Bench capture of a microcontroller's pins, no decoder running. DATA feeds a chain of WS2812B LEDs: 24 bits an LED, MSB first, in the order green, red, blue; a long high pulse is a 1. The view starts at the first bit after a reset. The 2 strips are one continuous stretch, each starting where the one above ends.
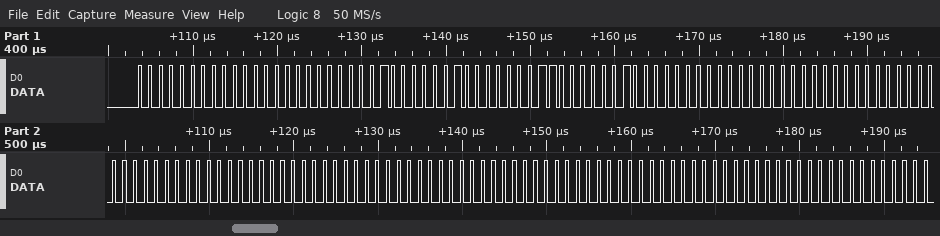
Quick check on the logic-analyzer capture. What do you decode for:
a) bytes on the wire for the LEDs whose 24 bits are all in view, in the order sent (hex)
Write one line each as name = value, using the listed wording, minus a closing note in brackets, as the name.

bytes on the wire for the LEDs whose 24 bits are all in view, in the order sent = 00 00 01 02 03 02 00 00 00 00 00 00 00 00 00 00 00 00
